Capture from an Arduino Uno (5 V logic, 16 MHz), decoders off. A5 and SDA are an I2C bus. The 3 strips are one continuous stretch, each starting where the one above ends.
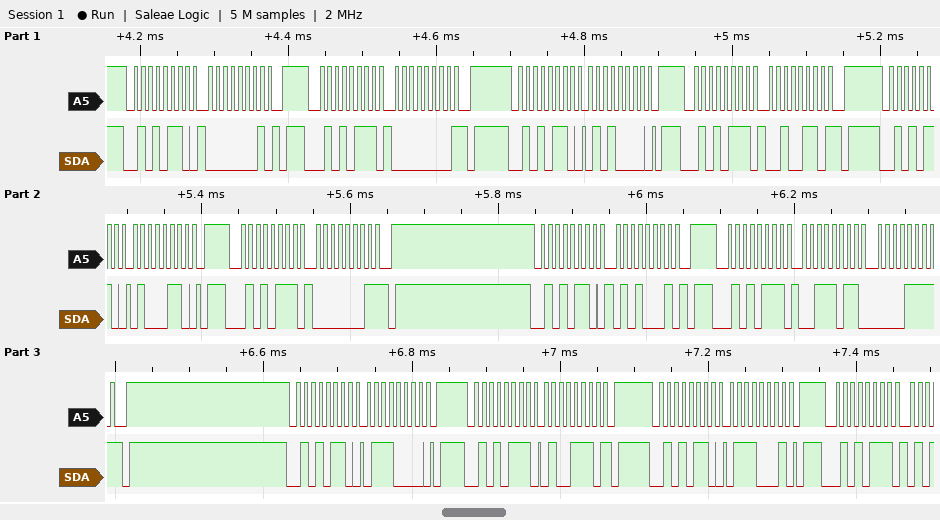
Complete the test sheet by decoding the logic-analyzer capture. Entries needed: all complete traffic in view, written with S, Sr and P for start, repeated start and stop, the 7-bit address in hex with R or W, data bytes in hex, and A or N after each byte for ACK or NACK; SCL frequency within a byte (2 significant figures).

S 2BW A 01 A P S 2BR A 00 N P S 2BW A 50 A P S 2BR A 26 N P S 2BW A 46 A P S 2BR A 01 N P S 2BW A 51 A P S 2BR A 3B A 0F N P S 2BW A 70 A P S 2BR A 4E N P S 2BW A 71 A P S 2BR A
100 kHz
